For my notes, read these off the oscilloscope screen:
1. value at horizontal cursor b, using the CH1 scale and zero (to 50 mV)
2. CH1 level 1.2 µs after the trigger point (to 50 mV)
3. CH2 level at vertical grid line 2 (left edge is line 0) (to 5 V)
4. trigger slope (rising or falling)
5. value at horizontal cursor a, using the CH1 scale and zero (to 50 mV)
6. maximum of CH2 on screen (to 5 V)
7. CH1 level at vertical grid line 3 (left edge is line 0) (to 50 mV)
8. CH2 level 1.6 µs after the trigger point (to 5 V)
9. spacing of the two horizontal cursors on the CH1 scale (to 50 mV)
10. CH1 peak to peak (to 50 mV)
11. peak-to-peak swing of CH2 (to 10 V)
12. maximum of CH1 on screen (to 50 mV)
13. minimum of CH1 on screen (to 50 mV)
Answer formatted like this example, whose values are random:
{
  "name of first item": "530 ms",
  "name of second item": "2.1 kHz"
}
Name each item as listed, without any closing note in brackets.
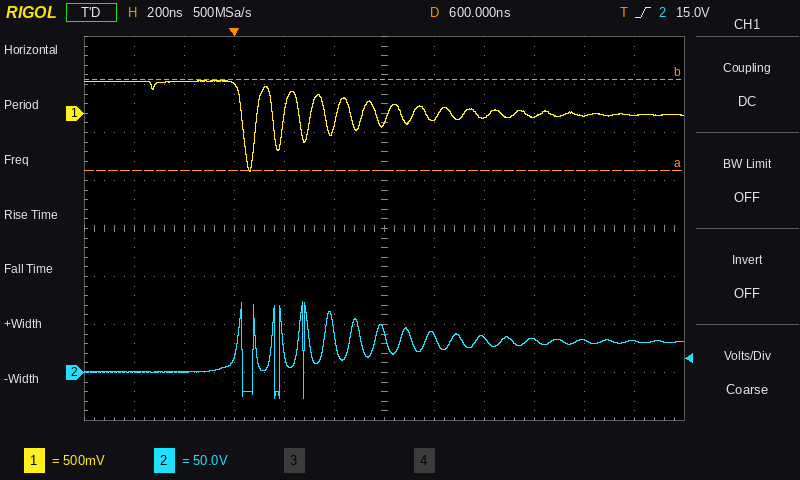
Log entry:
{
  "value at horizontal cursor b, using the CH1 scale and zero": "350 mV",
  "CH1 level 1.2 µs after the trigger point": "-50 mV",
  "CH2 level at vertical grid line 2 (left edge is line 0)": "0 V",
  "trigger slope": "rising",
  "value at horizontal cursor a, using the CH1 scale and zero": "-600 mV",
  "maximum of CH2 on screen": "75 V",
  "CH1 level at vertical grid line 3 (left edge is line 0)": "300 mV",
  "CH2 level 1.6 µs after the trigger point": "35 V",
  "spacing of the two horizontal cursors on the CH1 scale": "950 mV",
  "CH1 peak to peak": "950 mV",
  "peak-to-peak swing of CH2": "100 V",
  "maximum of CH1 on screen": "350 mV",
  "minimum of CH1 on screen": "-600 mV"
}
